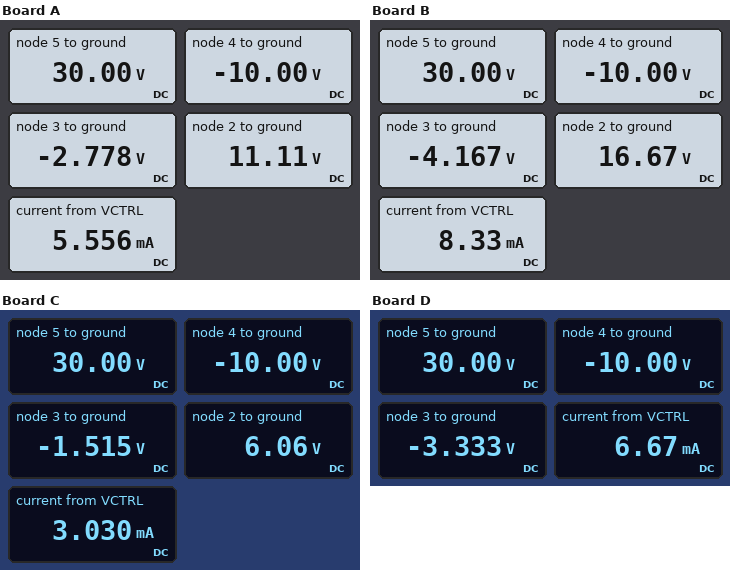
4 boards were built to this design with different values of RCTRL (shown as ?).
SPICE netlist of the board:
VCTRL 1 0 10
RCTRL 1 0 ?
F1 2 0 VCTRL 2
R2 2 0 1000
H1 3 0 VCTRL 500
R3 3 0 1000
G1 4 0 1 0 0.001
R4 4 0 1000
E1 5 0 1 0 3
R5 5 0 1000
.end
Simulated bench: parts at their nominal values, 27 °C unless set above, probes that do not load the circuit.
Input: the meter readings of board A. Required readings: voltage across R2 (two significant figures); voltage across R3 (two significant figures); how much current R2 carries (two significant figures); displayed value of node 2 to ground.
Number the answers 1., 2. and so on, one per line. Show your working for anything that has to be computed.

1. 11.11 V = 11 V
2. 0 V - (-2.778 V) = 2.8 V
3. (11.11 V) / 1 kΩ = 11 mA
4. 11.11 V
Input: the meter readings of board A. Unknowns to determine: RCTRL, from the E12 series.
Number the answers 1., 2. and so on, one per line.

1. 1.8 kΩ
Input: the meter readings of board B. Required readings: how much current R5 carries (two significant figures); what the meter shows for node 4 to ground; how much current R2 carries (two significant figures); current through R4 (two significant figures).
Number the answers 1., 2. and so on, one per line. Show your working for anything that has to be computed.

1. (30 V) / 1 kΩ = 30 mA
2. -10.00 V
3. (16.67 V) / 1 kΩ = 17 mA
4. (0 V - (-10 V)) / 1 kΩ = 10 mA
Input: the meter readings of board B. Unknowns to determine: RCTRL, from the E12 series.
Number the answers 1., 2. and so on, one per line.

1. 1.2 kΩ
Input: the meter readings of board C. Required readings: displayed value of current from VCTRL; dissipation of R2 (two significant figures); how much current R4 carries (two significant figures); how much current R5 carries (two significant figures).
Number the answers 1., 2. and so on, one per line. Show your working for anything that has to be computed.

1. 3.030 mA
2. (6.06 V)^2 / 1 kΩ = 37 mW
3. (0 V - (-10 V)) / 1 kΩ = 10 mA
4. (30 V) / 1 kΩ = 30 mA
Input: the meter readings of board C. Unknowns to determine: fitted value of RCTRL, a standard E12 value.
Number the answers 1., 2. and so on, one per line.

1. 3.3 kΩ
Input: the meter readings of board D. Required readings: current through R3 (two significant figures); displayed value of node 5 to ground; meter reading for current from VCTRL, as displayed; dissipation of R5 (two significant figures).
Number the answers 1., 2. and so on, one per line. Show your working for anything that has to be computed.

1. (0 V - (-3.333 V)) / 1 kΩ = 3.3 mA
2. 30.00 V
3. 6.67 mA
4. (30 V)^2 / 1 kΩ = 900 mW
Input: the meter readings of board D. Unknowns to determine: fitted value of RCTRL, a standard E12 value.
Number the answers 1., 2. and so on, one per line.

1. 1.5 kΩ
